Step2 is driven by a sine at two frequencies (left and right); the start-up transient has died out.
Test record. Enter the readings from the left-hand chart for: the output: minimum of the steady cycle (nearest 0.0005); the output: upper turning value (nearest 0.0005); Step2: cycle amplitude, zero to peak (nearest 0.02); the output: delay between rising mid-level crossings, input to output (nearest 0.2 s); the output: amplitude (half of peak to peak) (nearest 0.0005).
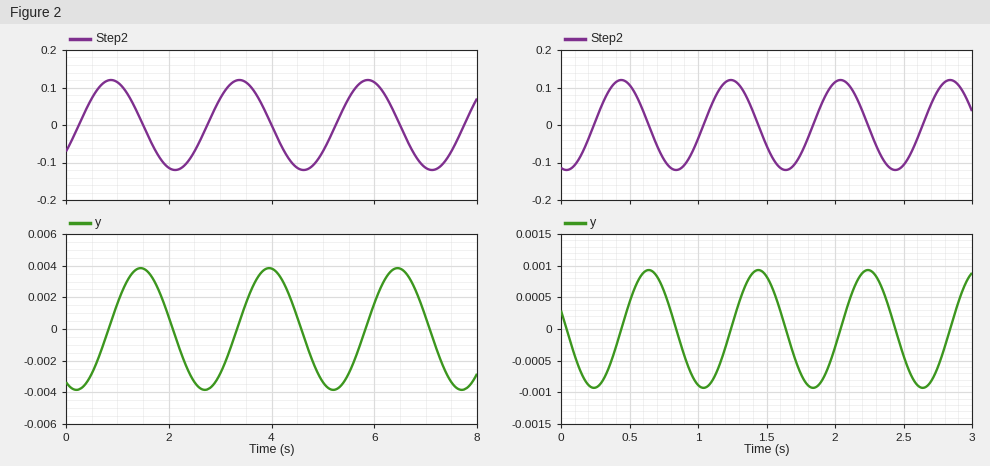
-0.0040
0.0040
0.12
0.6 s
0.0040
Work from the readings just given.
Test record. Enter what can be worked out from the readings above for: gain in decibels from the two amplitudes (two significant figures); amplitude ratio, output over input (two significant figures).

-30 dB
0.033
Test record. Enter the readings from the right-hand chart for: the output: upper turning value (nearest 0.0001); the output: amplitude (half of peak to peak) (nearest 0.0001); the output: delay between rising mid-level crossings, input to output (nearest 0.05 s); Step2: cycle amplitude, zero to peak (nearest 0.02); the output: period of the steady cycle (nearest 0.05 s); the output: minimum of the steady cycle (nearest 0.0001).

0.0009
0.0009
0.20 s
0.12
0.80 s
-0.0009
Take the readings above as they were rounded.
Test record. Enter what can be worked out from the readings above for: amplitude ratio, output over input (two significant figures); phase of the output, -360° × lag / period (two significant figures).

0.0075
-90°
